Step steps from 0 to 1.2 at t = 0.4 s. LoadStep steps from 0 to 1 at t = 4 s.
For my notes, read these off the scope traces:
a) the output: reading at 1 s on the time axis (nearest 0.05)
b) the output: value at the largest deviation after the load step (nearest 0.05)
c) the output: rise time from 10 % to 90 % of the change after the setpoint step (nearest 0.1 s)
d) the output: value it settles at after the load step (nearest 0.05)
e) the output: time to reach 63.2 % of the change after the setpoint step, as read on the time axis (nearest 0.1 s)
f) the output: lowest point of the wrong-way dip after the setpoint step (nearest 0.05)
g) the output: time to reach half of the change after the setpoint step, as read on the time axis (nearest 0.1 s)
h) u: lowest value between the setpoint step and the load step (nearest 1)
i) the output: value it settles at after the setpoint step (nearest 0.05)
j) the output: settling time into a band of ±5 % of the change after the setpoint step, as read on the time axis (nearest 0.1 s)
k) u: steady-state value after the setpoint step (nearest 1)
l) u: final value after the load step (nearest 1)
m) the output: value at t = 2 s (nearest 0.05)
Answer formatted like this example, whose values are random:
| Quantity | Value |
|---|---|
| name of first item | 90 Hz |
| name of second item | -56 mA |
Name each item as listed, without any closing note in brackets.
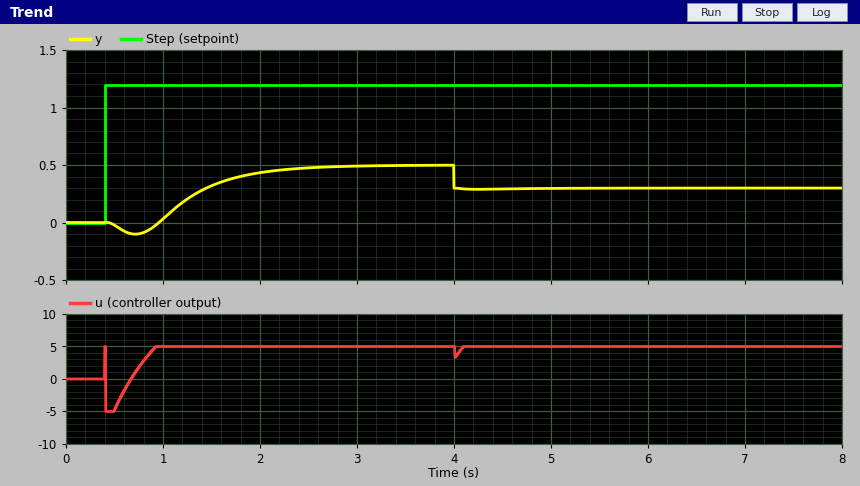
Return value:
| Quantity | Value |
|---|---|
| the output: reading at 1 s on the time axis | 0.05 |
| the output: value at the largest deviation after the load step | 0.30 |
| the output: rise time from 10 % to 90 % of the change after the setpoint step | 1.1 s |
| the output: value it settles at after the load step | 0.30 |
| the output: time to reach 63.2 % of the change after the setpoint step, as read on the time axis | 1.5 s |
| the output: lowest point of the wrong-way dip after the setpoint step | -0.10 |
| the output: time to reach half of the change after the setpoint step, as read on the time axis | 1.3 s |
| u: lowest value between the setpoint step and the load step | -5 |
| the output: value it settles at after the setpoint step | 0.50 |
| the output: settling time into a band of ±5 % of the change after the setpoint step, as read on the time axis | 2.5 s |
| u: steady-state value after the setpoint step | 5 |
| u: final value after the load step | 5 |
| the output: value at t = 2 s | 0.45 |
